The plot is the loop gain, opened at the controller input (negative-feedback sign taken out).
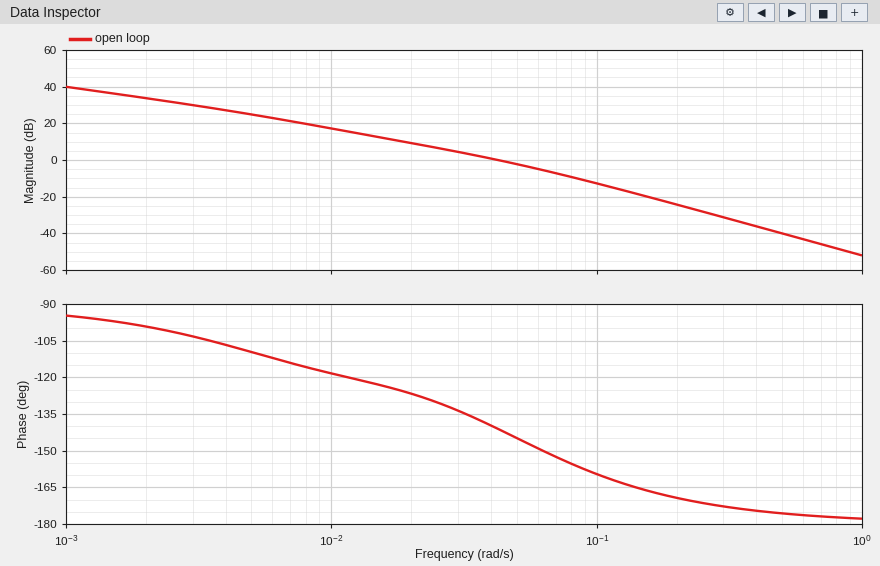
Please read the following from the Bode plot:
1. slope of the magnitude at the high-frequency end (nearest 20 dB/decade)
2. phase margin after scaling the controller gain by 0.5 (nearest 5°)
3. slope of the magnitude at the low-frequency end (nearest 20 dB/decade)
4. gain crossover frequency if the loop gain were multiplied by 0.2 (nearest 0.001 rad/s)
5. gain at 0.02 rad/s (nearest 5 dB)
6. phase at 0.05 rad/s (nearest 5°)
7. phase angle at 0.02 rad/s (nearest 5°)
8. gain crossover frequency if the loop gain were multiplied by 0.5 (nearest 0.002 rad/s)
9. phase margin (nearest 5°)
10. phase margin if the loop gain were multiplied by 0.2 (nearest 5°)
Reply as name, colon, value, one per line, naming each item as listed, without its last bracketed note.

slope of the magnitude at the high-frequency end: -40 dB/decade
phase margin after scaling the controller gain by 0.5: 50°
slope of the magnitude at the low-frequency end: -20 dB/decade
gain crossover frequency if the loop gain were multiplied by 0.2: 0.013 rad/s
gain at 0.02 rad/s: 10 dB
phase at 0.05 rad/s: -145°
phase angle at 0.02 rad/s: -125°
gain crossover frequency if the loop gain were multiplied by 0.5: 0.026 rad/s
phase margin: 40°
phase margin if the loop gain were multiplied by 0.2: 60°
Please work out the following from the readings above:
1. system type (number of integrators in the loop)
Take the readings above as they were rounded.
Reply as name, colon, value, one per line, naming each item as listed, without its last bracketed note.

system type: 1
